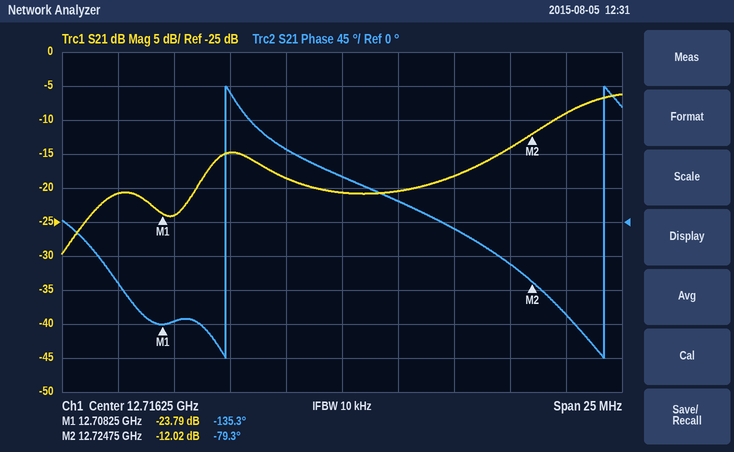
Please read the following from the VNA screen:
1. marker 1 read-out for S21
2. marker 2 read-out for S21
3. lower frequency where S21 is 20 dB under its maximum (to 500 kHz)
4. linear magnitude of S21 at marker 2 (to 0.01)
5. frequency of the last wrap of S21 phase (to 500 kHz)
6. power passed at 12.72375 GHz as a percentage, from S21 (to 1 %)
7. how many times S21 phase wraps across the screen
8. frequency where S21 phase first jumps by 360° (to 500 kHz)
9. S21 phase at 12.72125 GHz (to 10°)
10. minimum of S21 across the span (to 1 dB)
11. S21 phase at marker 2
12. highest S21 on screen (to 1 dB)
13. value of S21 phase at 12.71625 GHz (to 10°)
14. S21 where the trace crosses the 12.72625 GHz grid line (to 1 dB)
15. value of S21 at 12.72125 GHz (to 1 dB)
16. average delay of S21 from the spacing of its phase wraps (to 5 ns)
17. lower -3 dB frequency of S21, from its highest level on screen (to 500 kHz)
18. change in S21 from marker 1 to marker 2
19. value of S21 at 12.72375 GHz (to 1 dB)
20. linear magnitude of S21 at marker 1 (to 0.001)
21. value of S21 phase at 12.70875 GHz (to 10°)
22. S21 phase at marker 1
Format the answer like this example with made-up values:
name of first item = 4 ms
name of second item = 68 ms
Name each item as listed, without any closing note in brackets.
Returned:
marker 1 read-out for S21 = -23.79 dB
marker 2 read-out for S21 = -12.02 dB
lower frequency where S21 is 20 dB under its maximum = 12.7045 GHz
linear magnitude of S21 at marker 2 = 0.25
frequency of the last wrap of S21 phase = 12.7280 GHz
power passed at 12.72375 GHz as a percentage, from S21 = 4 %
how many times S21 phase wraps across the screen = 2
frequency where S21 phase first jumps by 360° = 12.7110 GHz
S21 phase at 12.72125 GHz = -10°
minimum of S21 across the span = -30 dB
S21 phase at marker 2 = -79.3°
highest S21 on screen = -6 dB
value of S21 phase at 12.71625 GHz = 60°
S21 where the trace crosses the 12.72625 GHz grid line = -9 dB
value of S21 at 12.72125 GHz = -18 dB
average delay of S21 from the spacing of its phase wraps = 60 ns
lower -3 dB frequency of S21, from its highest level on screen = 12.7260 GHz
change in S21 from marker 1 to marker 2 = 11.77 dB
value of S21 at 12.72375 GHz = -14 dB
linear magnitude of S21 at marker 1 = 0.065
value of S21 phase at 12.70875 GHz = -130°
S21 phase at marker 1 = -135.3°
